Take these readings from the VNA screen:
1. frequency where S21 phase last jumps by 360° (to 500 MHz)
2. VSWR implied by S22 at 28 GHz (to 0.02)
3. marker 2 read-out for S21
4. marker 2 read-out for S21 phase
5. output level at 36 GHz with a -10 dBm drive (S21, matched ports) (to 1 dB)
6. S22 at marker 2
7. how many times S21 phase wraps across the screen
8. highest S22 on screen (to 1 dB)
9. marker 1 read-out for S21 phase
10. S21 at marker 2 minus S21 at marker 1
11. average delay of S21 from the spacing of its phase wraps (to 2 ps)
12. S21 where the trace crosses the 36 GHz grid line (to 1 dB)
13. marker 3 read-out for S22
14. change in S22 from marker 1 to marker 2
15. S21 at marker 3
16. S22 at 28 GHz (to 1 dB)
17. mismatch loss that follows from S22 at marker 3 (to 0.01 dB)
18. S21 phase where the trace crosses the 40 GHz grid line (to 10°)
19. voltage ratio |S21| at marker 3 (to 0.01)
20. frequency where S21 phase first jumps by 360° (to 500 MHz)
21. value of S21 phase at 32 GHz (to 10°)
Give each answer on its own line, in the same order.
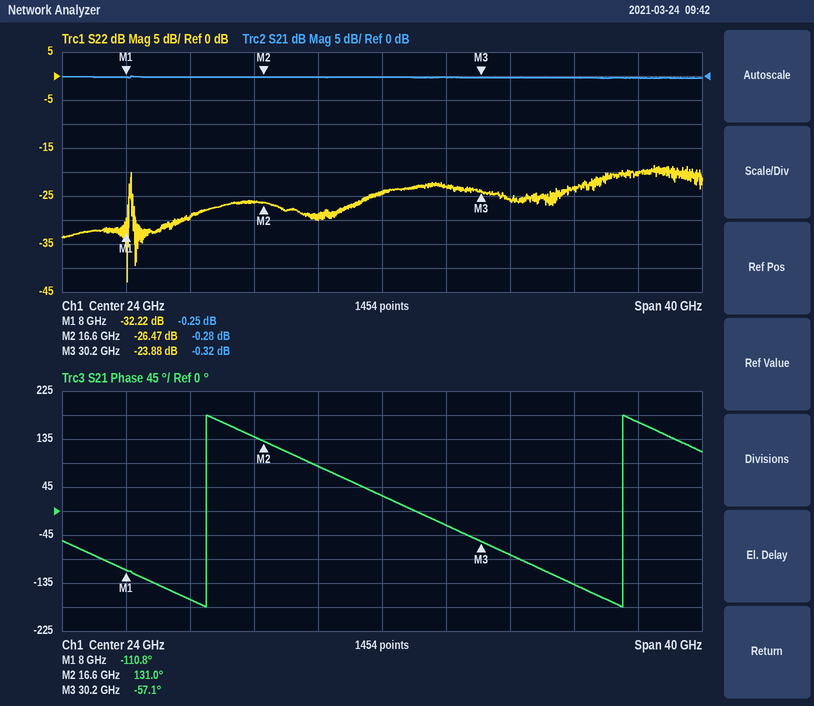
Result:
39.0 GHz
1.16
-0.28 dB
131.0°
-10 dBm
-26.47 dB
2
-19 dB
-110.8°
-0.03 dB
38 ps
0 dB
-23.88 dB
5.75 dB
-0.32 dB
-23 dB
0.02 dB
170°
0.96
13.0 GHz
-80°
